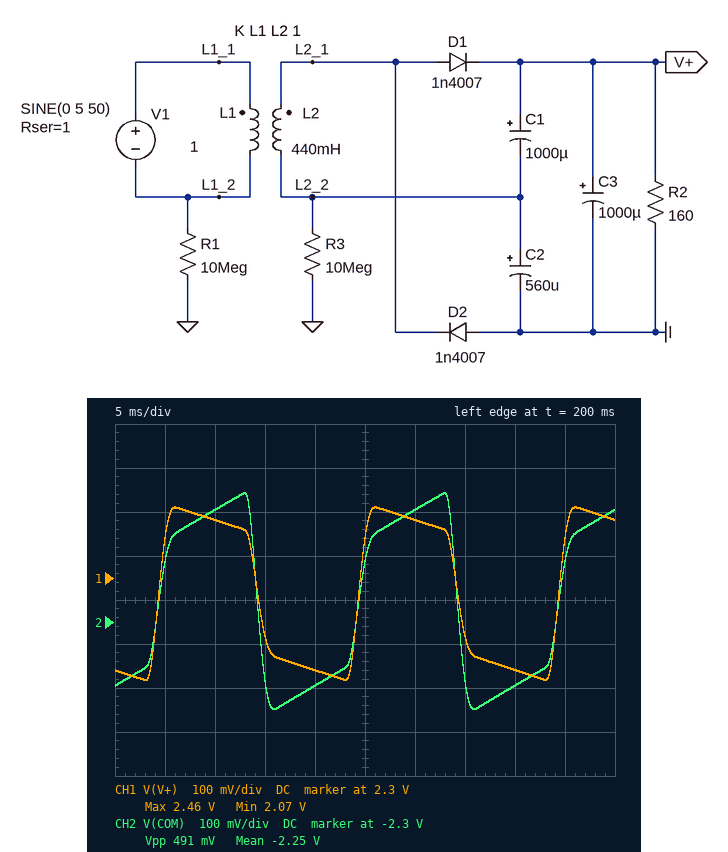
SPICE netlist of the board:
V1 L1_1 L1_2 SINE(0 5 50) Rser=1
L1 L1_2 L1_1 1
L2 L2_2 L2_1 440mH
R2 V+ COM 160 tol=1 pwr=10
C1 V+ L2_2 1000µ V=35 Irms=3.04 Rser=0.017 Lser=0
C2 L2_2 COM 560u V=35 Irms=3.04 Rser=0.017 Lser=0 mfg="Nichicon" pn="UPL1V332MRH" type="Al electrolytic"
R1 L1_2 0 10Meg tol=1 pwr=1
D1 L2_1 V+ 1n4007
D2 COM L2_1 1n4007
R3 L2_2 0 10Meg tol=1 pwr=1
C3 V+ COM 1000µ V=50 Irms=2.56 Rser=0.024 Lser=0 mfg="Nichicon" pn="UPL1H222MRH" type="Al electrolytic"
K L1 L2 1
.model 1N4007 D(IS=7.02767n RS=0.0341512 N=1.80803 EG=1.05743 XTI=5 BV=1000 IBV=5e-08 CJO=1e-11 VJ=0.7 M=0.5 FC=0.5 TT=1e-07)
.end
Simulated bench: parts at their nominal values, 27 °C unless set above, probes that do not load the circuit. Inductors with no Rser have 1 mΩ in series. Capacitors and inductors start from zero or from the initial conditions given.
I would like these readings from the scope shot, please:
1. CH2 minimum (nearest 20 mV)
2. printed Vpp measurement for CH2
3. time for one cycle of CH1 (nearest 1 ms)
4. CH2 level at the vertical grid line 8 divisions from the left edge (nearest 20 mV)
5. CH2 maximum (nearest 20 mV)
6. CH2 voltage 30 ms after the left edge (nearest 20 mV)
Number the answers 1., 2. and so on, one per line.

1. -2.50 V
2. 491 mV
3. 20 ms
4. -2.44 V
5. -2.00 V
6. -2.04 V
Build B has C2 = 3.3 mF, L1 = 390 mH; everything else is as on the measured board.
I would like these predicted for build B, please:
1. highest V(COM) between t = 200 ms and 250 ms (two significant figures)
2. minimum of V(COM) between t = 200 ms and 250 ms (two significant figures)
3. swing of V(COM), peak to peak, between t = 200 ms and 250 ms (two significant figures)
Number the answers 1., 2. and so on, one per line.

1. -3.8 V
2. -4.1 V
3. 240 mV
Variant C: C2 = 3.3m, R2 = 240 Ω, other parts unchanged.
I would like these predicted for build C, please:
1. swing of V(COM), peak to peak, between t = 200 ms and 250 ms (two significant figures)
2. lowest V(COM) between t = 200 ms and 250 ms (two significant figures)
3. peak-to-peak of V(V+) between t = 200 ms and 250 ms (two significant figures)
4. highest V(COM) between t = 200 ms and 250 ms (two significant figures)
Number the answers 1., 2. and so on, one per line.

1. 97 mV
2. -2.4 V
3. 200 mV
4. -2.3 V
